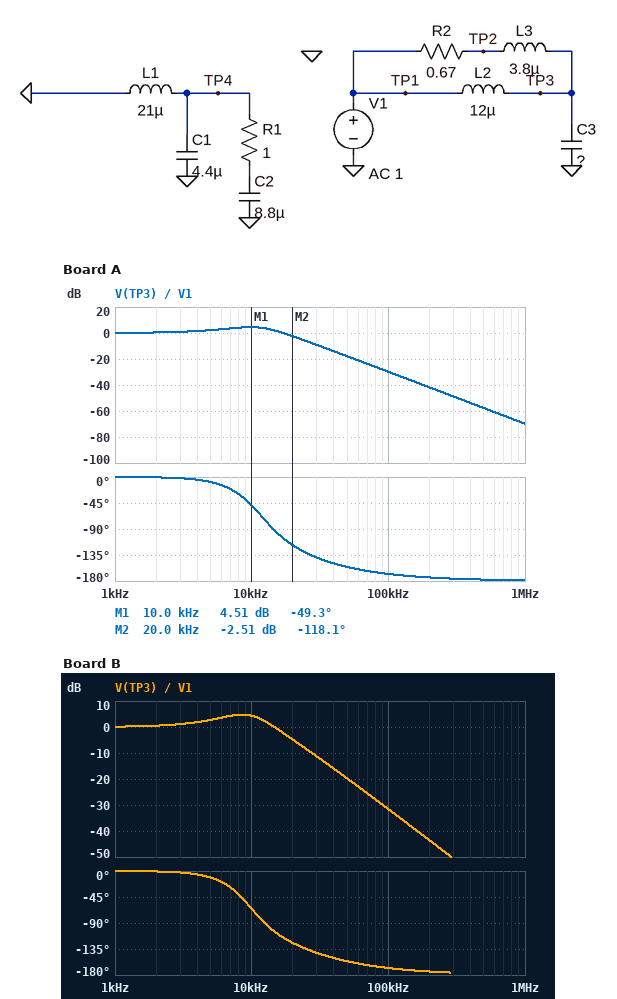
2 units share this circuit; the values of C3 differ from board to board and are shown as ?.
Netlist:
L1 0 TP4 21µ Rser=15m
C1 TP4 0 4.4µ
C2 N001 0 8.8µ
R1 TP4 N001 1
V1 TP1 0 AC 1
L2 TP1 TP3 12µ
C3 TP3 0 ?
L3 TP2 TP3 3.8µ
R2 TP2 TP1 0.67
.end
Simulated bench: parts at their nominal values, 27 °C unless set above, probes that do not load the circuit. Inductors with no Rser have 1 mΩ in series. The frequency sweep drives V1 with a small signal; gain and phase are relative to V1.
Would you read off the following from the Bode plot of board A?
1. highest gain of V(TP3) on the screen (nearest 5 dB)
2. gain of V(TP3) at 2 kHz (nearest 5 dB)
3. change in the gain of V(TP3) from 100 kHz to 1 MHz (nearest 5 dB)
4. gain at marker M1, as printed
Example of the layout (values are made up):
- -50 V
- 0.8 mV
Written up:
- 5 dB
- 0 dB
- -40 dB
- 4.51 dB
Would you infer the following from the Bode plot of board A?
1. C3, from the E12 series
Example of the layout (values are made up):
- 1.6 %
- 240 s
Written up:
- 27 µF
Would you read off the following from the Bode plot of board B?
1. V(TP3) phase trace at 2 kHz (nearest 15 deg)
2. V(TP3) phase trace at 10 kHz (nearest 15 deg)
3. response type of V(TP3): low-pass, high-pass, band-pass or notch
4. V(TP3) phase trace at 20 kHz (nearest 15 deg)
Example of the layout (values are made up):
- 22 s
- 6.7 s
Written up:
- 0 deg
- -60 deg
- low-pass
- -120 deg
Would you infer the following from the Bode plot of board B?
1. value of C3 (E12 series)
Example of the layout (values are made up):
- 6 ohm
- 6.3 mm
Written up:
- 33 µF
